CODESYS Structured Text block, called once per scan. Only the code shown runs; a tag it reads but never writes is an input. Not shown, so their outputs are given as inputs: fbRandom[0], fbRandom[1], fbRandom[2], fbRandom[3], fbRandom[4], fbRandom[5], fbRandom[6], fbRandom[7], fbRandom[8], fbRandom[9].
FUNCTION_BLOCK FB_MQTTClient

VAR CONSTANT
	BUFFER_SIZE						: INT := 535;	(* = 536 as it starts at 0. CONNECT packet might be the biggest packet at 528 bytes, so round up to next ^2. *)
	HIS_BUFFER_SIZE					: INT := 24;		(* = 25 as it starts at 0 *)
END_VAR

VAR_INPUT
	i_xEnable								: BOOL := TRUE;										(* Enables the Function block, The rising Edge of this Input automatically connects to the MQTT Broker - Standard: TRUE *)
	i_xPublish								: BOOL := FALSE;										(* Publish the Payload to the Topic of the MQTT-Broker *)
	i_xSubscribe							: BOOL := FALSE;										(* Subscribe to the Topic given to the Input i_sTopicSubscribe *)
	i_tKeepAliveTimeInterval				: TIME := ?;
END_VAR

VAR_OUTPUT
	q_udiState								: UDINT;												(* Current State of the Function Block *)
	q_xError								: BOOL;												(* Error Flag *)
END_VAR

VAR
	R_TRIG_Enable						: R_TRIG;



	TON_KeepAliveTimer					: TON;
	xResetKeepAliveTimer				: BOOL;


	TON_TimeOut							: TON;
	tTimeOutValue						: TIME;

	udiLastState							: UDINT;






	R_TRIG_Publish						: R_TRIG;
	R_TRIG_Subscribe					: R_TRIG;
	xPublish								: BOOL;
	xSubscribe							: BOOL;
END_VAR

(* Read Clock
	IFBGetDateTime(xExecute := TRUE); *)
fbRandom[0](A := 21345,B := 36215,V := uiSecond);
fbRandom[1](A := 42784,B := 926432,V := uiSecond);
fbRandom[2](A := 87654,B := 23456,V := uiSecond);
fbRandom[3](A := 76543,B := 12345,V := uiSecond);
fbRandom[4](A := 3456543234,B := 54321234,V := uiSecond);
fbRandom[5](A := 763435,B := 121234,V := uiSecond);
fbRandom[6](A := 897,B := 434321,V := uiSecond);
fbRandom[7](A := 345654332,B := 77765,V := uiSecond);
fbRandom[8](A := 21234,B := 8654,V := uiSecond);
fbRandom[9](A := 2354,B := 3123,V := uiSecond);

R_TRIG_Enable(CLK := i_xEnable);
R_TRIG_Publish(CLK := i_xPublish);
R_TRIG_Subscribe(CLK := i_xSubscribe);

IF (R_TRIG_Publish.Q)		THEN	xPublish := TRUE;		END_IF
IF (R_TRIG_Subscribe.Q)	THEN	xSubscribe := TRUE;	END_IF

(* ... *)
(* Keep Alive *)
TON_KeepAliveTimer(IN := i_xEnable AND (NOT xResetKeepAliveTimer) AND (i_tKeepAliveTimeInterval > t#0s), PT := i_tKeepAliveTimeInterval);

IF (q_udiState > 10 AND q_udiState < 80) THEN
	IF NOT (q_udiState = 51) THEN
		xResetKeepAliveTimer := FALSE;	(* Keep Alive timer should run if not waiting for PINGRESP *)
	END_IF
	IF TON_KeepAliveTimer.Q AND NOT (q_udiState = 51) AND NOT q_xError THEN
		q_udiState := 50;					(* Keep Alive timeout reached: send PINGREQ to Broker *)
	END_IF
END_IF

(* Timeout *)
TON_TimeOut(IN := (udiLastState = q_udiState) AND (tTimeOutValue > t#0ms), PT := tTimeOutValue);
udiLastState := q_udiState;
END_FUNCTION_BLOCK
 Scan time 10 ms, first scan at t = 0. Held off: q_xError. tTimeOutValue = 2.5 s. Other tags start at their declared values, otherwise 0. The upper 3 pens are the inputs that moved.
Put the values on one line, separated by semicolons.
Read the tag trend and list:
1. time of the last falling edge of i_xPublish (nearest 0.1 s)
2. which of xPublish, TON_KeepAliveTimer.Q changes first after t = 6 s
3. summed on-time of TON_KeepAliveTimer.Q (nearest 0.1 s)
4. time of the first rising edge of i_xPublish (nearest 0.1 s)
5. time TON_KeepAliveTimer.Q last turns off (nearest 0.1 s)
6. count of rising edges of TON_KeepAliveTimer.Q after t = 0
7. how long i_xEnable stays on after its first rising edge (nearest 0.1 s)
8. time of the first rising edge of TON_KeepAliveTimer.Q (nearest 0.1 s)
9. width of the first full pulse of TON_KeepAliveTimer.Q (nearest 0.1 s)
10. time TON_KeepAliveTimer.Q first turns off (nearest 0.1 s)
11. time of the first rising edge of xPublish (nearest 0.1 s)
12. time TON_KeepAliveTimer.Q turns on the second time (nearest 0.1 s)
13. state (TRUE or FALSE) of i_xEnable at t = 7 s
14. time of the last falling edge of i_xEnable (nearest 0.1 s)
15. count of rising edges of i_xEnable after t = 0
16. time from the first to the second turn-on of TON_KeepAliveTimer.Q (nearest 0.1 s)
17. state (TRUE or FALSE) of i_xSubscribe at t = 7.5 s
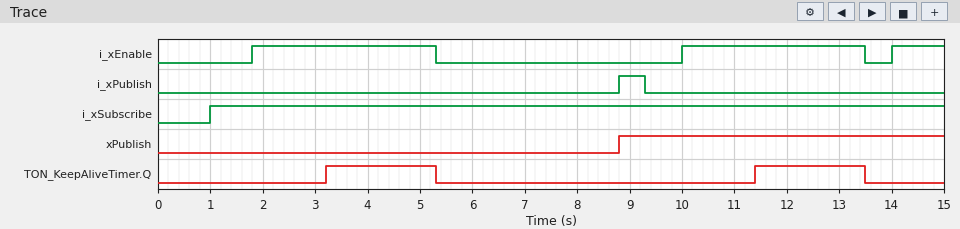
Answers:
9.3 s; xPublish; 4.2 s; 8.8 s; 13.5 s; 2; 3.5 s; 3.2 s; 2.1 s; 5.3 s; 8.8 s; 11.4 s; FALSE; 13.5 s; 3; 8.2 s; TRUE
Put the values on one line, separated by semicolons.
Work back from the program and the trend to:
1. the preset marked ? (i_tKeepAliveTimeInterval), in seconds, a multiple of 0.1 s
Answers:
1.4 s
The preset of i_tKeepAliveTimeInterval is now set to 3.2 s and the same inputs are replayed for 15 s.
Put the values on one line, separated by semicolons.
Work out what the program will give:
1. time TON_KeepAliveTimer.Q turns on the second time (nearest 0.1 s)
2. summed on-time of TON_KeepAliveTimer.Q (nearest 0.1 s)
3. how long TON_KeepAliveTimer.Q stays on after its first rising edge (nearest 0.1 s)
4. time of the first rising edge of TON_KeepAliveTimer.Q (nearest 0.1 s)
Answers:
13.2 s; 0.6 s; 0.3 s; 5.0 s
